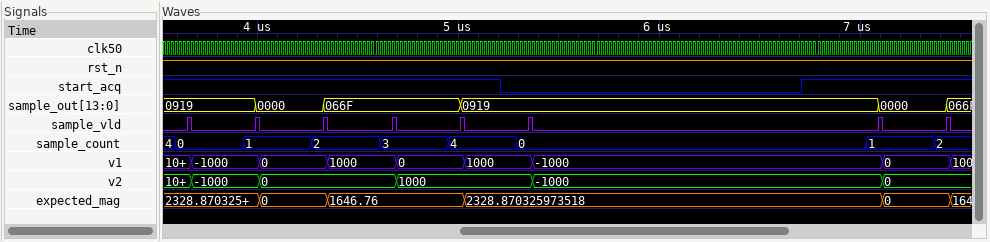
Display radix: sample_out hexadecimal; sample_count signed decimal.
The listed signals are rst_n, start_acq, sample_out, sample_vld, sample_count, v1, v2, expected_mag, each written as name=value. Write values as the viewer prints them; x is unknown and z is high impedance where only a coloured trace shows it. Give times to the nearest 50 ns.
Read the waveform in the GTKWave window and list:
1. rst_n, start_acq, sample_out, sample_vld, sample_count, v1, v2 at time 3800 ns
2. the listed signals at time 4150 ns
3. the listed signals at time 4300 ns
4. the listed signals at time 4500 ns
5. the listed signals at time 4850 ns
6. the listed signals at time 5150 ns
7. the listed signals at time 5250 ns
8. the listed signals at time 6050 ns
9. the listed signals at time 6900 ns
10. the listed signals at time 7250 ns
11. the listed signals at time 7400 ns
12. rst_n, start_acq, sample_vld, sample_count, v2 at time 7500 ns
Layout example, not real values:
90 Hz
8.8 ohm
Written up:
rst_n=1, start_acq=1, sample_out=0919, sample_vld=0, sample_count=0, v1=-1000, v2=-1000
rst_n=1, start_acq=1, sample_out=0000, sample_vld=0, sample_count=1, v1=0, v2=0, expected_mag=0
rst_n=1, start_acq=1, sample_out=0000, sample_vld=0, sample_count=2, v1=0, v2=0, expected_mag=0
rst_n=1, start_acq=1, sample_out=066F, sample_vld=0, sample_count=2, v1=1000, v2=0, expected_mag=1646.76
rst_n=1, start_acq=1, sample_out=066F, sample_vld=0, sample_count=3, v1=0, v2=1000, expected_mag=1646.76
rst_n=1, start_acq=1, sample_out=0919, sample_vld=0, sample_count=4, v1=1000, v2=1000, expected_mag=2328.870325973518
rst_n=1, start_acq=0, sample_out=0919, sample_vld=0, sample_count=4, v1=1000, v2=1000, expected_mag=2328.870325973518
rst_n=1, start_acq=0, sample_out=0919, sample_vld=0, sample_count=0, v1=-1000, v2=-1000, expected_mag=2328.870325973518
rst_n=1, start_acq=1, sample_out=0919, sample_vld=0, sample_count=0, v1=-1000, v2=-1000, expected_mag=2328.870325973518
rst_n=1, start_acq=1, sample_out=0000, sample_vld=0, sample_count=1, v1=0, v2=0, expected_mag=0
rst_n=1, start_acq=1, sample_out=0000, sample_vld=0, sample_count=2, v1=0, v2=0, expected_mag=0
rst_n=1, start_acq=1, sample_vld=0, sample_count=2, v2=0
